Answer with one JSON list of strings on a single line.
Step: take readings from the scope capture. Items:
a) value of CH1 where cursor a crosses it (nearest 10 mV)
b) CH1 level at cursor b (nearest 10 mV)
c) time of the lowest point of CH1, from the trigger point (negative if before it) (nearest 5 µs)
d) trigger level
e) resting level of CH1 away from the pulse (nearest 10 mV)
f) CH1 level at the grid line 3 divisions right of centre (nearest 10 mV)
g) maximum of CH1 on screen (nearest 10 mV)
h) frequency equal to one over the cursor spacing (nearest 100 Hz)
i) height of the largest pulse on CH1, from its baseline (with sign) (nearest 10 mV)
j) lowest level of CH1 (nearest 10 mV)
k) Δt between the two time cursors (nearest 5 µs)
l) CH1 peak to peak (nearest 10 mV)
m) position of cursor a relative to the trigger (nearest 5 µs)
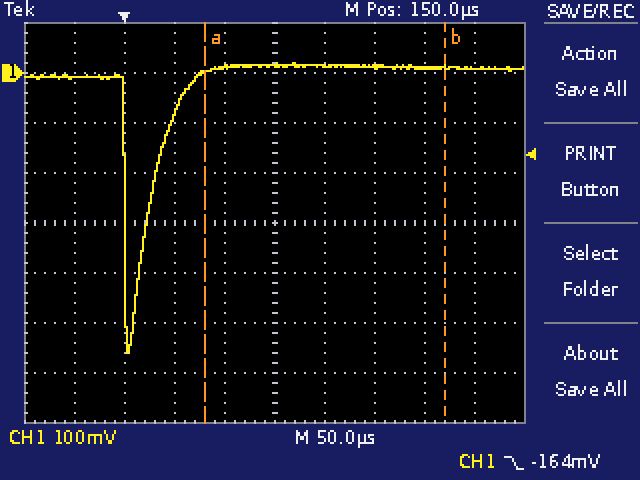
["0 mV", "10 mV", "+5 µs", "-164 mV", "10 mV", "10 mV", "20 mV", "4.2 kHz", "-570 mV", "-560 mV", "240 µs", "580 mV", "+80 µs"]
